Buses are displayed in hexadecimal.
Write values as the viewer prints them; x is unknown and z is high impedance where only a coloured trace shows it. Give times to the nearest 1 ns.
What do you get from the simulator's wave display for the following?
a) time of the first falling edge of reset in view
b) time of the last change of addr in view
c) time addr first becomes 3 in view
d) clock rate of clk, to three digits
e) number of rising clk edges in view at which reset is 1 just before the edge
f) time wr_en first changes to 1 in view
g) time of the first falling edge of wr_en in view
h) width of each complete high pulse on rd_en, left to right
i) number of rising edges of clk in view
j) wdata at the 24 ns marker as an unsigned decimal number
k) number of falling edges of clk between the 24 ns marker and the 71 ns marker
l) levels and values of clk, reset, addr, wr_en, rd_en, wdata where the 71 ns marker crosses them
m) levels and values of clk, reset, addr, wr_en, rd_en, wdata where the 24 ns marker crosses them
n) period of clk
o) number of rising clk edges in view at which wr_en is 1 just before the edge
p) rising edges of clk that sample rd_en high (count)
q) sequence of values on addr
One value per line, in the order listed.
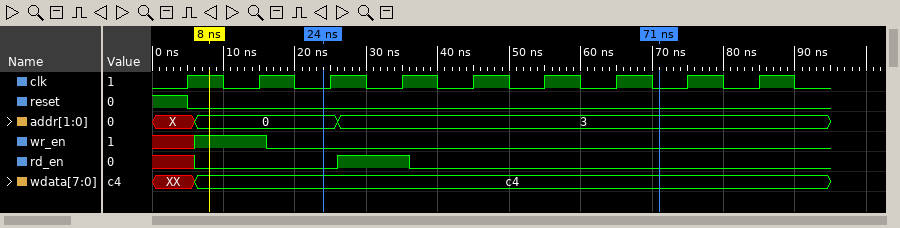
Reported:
5 ns
26 ns
26 ns
100 MHz
1
6 ns
16 ns
10 ns
9
196
5
clk=0, reset=0, addr=3, wr_en=0, rd_en=0, wdata=c4
clk=0, reset=0, addr=0, wr_en=0, rd_en=0, wdata=c4
10 ns
1
1
X, 0, 3
